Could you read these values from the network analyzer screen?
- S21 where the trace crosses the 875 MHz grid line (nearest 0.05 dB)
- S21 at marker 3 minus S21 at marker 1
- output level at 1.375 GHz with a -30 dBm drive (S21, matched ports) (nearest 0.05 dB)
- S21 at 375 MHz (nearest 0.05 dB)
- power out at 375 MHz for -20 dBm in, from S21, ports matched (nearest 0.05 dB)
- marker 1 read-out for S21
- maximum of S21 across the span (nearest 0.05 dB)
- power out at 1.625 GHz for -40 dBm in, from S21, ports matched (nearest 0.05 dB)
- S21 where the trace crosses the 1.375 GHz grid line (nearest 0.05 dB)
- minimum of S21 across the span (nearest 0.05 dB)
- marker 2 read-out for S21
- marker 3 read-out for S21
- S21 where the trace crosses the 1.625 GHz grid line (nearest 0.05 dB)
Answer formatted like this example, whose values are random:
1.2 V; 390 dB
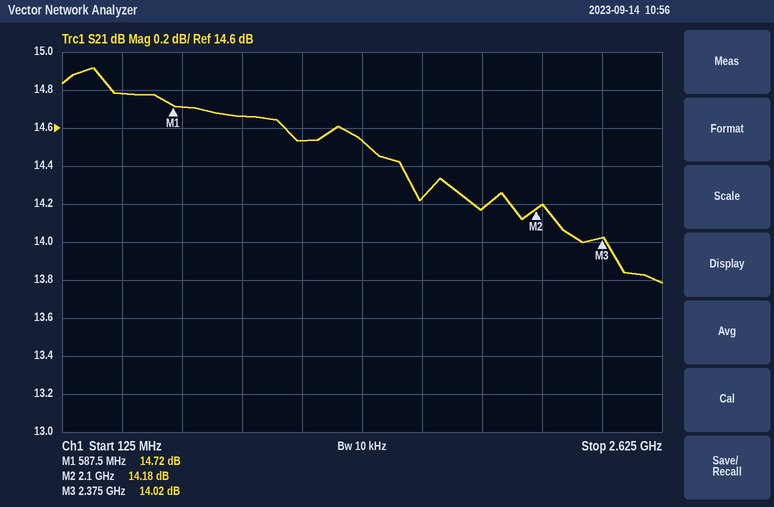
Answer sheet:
14.65 dB; -0.70 dB; -15.45 dBm; 14.80 dB; -5.20 dBm; 14.72 dB; 14.90 dB; -25.75 dBm; 14.55 dB; 13.80 dB; 14.18 dB; 14.02 dB; 14.25 dB
